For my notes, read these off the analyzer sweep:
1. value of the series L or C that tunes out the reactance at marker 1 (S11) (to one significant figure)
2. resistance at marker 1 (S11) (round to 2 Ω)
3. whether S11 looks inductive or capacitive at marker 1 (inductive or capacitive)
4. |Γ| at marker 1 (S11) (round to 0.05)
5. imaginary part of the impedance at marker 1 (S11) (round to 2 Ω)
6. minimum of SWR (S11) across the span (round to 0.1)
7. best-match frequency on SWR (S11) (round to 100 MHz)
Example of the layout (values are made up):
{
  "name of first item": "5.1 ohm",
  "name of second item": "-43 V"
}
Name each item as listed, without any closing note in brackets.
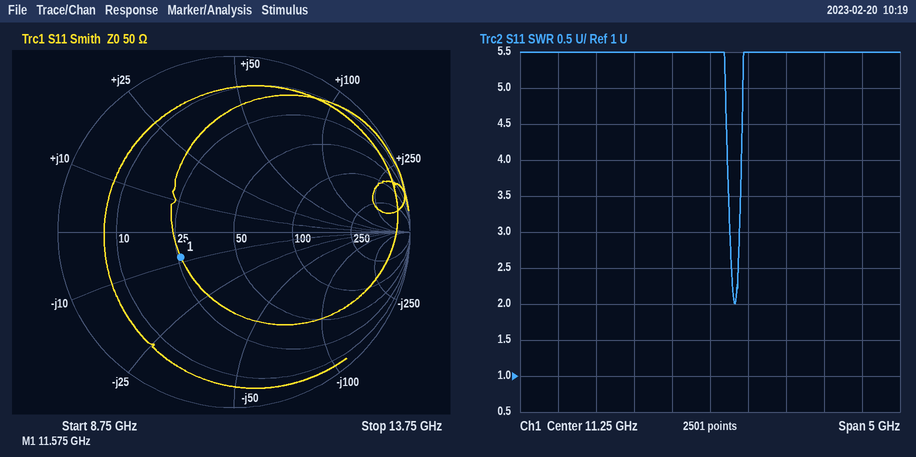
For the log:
{
  "value of the series L or C that tunes out the reactance at marker 1 (S11)": "100 pH",
  "resistance at marker 1 (S11)": "26 Ω",
  "whether S11 looks inductive or capacitive at marker 1": "capacitive",
  "|Γ| at marker 1 (S11)": "0.35",
  "imaginary part of the impedance at marker 1 (S11)": "-8 Ω",
  "minimum of SWR (S11) across the span": "2.0",
  "best-match frequency on SWR (S11)": "11.6 GHz"
}
